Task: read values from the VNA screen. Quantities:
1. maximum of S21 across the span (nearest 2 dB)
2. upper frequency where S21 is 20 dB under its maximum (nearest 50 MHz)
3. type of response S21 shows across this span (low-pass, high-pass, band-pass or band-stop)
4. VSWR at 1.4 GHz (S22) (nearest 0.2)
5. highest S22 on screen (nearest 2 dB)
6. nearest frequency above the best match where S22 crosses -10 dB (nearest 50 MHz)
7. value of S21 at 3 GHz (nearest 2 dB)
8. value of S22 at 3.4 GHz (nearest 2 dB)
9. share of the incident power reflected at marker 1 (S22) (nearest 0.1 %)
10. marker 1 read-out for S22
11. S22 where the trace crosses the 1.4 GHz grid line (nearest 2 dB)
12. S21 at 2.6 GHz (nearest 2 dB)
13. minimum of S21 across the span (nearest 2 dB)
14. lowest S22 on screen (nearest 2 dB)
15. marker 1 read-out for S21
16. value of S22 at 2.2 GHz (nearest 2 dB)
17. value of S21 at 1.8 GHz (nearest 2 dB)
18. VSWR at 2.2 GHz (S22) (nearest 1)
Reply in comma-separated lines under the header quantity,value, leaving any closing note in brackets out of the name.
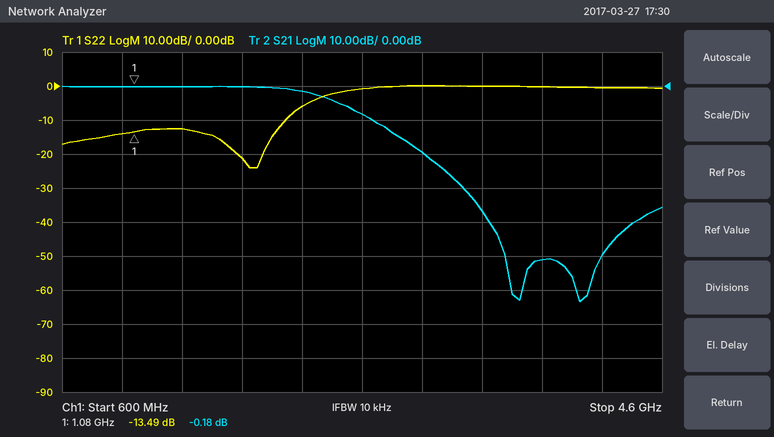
quantity,value
maximum of S21 across the span,0 dB
upper frequency where S21 is 20 dB under its maximum,3.00 GHz
type of response S21 shows across this span,low-pass
VSWR at 1.4 GHz (S22),1.6
highest S22 on screen,0 dB
nearest frequency above the best match where S22 crosses -10 dB,2.10 GHz
value of S21 at 3 GHz,-20 dB
value of S22 at 3.4 GHz,0 dB
share of the incident power reflected at marker 1 (S22),4.5 %
marker 1 read-out for S22,-13.49 dB
S22 where the trace crosses the 1.4 GHz grid line,-12 dB
S21 at 2.6 GHz,-8 dB
minimum of S21 across the span,-64 dB
lowest S22 on screen,-24 dB
marker 1 read-out for S21,-0.18 dB
value of S22 at 2.2 GHz,-6 dB
value of S21 at 1.8 GHz,0 dB
VSWR at 2.2 GHz (S22),3
